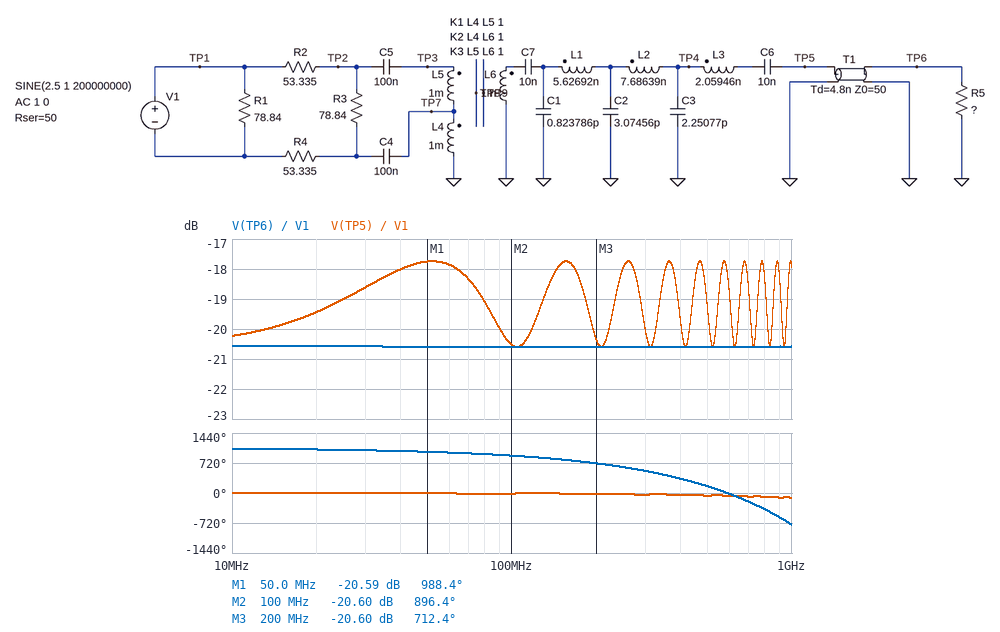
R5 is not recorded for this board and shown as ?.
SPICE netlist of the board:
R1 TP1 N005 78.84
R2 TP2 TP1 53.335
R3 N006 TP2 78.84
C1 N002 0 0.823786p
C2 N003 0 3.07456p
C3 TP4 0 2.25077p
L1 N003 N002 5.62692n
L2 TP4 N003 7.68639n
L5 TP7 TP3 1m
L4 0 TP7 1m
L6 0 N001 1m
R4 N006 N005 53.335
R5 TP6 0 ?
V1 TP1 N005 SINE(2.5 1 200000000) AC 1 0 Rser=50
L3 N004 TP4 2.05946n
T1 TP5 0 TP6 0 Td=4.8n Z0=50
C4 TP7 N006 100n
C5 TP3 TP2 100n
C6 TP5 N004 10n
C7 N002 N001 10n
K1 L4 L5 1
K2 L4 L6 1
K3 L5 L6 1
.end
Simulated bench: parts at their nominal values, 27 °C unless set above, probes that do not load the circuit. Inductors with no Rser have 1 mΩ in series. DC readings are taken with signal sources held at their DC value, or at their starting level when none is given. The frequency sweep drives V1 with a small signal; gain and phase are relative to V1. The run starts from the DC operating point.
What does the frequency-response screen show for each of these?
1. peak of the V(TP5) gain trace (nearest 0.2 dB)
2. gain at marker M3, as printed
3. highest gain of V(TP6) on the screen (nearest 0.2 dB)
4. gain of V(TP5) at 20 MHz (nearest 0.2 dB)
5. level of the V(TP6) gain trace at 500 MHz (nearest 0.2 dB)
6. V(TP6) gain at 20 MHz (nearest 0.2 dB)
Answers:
-17.8 dB
-20.60 dB
-20.6 dB
-19.4 dB
-20.6 dB
-20.6 dB
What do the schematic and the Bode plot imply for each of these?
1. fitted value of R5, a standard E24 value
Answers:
36 Ω
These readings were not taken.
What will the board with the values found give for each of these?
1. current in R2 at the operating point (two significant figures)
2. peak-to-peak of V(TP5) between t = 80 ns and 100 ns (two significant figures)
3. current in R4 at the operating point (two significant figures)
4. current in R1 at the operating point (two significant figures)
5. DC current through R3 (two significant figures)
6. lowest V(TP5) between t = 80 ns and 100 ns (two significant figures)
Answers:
7.1 mA
190 mV
7.1 mA
17 mA
7.1 mA
-96 mV
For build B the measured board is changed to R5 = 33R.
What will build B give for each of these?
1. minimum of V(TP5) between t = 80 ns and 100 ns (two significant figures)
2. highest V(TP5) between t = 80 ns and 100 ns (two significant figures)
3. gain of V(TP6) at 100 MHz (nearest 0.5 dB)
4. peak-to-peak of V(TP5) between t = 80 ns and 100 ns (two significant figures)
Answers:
-92 mV
92 mV
-21.0 dB
180 mV
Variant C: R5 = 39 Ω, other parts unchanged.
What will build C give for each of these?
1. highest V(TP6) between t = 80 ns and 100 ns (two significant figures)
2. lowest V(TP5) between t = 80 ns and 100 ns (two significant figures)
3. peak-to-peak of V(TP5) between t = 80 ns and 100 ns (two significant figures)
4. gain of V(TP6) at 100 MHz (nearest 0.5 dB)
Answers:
98 mV
-100 mV
200 mV
-20.0 dB
